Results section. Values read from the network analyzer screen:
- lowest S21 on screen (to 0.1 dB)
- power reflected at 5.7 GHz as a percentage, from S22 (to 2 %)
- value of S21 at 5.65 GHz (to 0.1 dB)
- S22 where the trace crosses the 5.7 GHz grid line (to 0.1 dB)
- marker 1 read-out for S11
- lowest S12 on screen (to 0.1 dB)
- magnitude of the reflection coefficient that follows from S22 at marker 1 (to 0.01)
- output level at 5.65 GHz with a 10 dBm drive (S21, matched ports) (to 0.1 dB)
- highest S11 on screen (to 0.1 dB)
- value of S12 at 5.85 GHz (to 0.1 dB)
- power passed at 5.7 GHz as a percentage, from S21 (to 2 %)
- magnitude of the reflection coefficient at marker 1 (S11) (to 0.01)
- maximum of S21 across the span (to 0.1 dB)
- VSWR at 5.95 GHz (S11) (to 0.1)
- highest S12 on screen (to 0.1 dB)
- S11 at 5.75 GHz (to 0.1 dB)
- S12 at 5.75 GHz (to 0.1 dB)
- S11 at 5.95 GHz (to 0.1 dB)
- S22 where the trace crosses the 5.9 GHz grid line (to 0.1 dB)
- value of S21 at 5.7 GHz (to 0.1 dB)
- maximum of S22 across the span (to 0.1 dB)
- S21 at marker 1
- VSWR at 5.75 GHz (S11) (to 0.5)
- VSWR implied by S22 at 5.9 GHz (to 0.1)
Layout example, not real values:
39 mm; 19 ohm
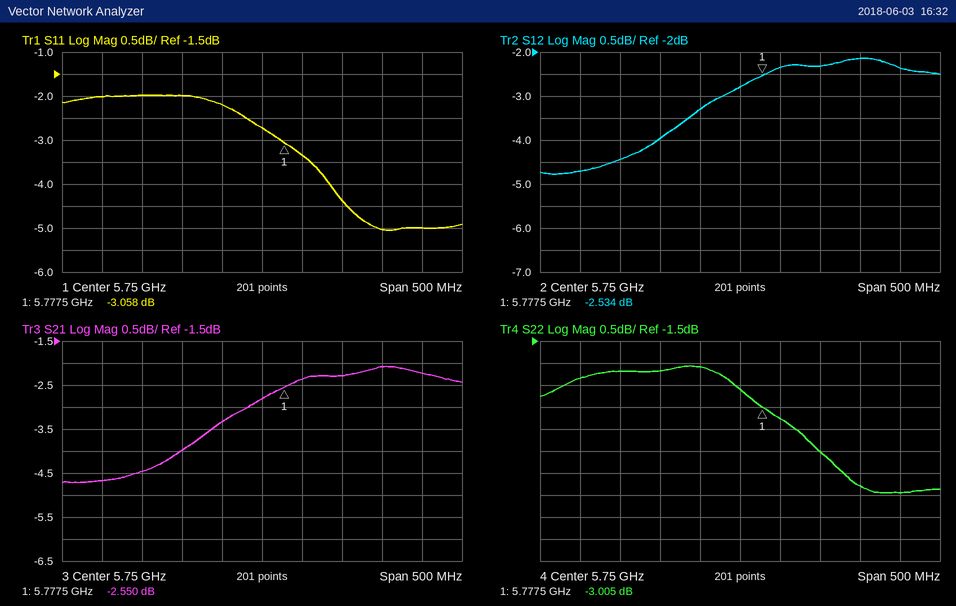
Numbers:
-4.7 dB; 62 %; -4.0 dB; -2.1 dB; -3.058 dB; -4.8 dB; 0.71; 6.0 dBm; -2.0 dB; -2.3 dB; 46 %; 0.70; -2.1 dB; 3.6; -2.1 dB; -2.7 dB; -2.8 dB; -5.0 dB; -4.8 dB; -3.3 dB; -2.1 dB; -2.550 dB; 6.5; 3.7
